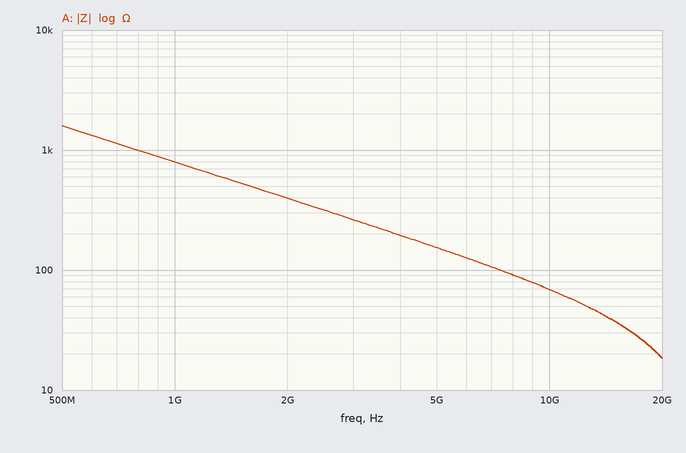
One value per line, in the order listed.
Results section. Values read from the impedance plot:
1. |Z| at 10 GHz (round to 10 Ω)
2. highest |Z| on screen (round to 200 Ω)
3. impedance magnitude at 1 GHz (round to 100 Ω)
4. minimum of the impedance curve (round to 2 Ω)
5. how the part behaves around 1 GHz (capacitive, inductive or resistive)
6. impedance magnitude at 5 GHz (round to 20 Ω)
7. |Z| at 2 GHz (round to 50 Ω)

70 Ω
1.6 kΩ
800 Ω
18 Ω
capacitive
160 Ω
400 Ω
